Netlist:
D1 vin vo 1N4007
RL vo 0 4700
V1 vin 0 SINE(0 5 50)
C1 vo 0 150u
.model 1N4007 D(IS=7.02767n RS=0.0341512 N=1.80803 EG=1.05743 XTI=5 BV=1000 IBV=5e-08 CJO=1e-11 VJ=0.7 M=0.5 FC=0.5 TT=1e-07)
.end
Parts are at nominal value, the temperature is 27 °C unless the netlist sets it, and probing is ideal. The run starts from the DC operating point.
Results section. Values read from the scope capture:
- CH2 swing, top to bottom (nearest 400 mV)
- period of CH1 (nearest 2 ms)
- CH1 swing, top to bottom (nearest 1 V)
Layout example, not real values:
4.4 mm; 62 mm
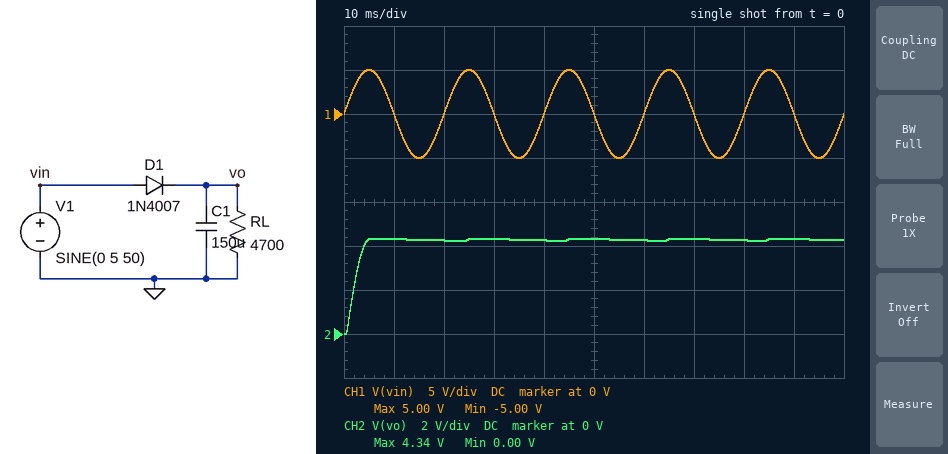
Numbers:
4.4 V; 20 ms; 10 V
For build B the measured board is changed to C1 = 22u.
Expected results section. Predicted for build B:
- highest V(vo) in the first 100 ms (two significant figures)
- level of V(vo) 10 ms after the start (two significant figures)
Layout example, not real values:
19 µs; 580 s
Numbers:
4.4 V; 4.2 V
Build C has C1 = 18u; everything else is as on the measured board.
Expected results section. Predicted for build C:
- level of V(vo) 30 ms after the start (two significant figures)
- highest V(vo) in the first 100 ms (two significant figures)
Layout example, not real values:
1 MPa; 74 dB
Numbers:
4.2 V; 4.4 V
